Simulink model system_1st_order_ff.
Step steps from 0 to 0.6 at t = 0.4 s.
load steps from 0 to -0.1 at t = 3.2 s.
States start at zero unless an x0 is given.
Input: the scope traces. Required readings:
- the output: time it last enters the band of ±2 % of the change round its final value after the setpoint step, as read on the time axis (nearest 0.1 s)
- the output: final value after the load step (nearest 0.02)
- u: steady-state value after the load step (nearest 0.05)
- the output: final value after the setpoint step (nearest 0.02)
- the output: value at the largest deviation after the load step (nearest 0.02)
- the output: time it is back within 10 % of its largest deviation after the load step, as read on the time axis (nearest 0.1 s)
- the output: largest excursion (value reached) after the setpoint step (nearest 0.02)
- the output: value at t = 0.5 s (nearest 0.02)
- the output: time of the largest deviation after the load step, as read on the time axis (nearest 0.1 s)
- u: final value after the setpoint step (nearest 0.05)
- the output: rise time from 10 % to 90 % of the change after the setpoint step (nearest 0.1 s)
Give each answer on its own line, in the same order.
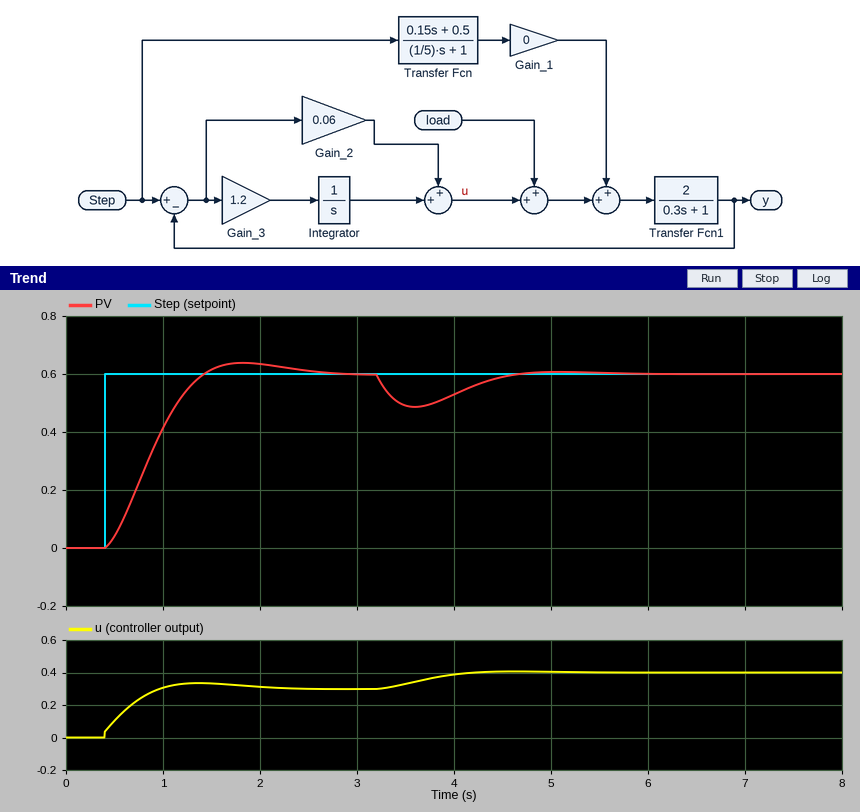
2.5 s
0.60
0.40
0.60
0.48
4.5 s
0.64
0.04
3.6 s
0.30
0.7 s
